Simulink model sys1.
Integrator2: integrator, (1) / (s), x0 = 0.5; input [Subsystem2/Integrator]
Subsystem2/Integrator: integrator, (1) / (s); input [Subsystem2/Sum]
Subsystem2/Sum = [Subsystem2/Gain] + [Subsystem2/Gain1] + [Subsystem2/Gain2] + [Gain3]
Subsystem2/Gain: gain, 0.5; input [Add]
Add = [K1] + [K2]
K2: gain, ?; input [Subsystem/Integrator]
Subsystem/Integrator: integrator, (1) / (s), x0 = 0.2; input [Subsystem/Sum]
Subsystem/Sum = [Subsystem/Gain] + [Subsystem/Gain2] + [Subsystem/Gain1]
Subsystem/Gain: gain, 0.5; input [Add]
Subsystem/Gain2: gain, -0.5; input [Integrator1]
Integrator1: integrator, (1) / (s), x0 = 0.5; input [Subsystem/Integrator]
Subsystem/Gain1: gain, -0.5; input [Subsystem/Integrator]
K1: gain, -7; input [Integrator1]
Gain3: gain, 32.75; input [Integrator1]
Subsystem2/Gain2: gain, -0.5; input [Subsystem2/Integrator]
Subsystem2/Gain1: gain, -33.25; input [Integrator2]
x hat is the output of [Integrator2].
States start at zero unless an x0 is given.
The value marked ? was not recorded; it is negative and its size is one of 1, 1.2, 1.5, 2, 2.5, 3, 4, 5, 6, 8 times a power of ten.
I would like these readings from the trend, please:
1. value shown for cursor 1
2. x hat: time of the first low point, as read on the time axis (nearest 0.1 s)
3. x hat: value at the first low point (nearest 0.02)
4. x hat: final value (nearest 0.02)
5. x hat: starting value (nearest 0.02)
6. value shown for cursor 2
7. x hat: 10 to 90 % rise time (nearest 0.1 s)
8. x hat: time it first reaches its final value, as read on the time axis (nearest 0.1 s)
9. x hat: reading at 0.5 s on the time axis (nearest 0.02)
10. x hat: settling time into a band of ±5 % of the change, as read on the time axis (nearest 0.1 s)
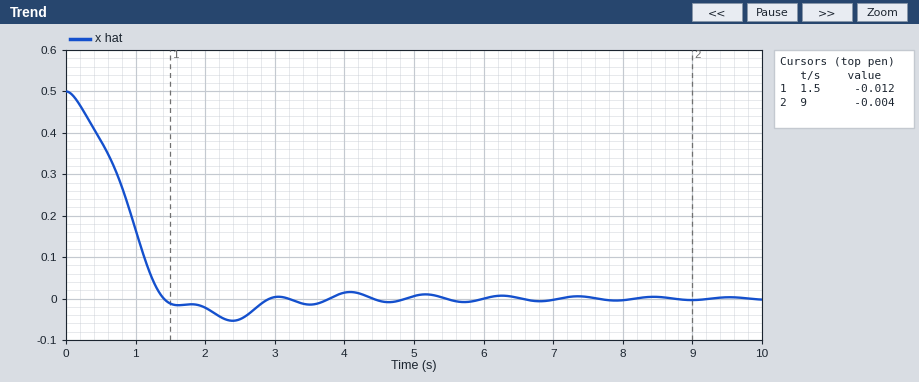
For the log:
-0.012
2.4 s
-0.06
0.00
0.50
-0.004
1.0 s
1.4 s
0.38
2.7 s
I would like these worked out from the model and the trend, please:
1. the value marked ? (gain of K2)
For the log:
-4
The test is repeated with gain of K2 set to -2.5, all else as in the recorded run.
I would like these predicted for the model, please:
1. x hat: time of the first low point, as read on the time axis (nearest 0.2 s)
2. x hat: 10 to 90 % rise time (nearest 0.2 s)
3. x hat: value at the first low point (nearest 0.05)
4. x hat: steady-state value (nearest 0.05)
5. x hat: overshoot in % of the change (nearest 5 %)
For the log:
1.6 s
0.8 s
-0.10
0.00
20 %
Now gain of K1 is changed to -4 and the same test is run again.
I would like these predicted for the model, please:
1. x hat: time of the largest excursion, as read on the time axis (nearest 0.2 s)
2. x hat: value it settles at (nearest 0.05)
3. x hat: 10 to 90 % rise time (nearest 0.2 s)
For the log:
3.6 s
0.00
1.6 s
